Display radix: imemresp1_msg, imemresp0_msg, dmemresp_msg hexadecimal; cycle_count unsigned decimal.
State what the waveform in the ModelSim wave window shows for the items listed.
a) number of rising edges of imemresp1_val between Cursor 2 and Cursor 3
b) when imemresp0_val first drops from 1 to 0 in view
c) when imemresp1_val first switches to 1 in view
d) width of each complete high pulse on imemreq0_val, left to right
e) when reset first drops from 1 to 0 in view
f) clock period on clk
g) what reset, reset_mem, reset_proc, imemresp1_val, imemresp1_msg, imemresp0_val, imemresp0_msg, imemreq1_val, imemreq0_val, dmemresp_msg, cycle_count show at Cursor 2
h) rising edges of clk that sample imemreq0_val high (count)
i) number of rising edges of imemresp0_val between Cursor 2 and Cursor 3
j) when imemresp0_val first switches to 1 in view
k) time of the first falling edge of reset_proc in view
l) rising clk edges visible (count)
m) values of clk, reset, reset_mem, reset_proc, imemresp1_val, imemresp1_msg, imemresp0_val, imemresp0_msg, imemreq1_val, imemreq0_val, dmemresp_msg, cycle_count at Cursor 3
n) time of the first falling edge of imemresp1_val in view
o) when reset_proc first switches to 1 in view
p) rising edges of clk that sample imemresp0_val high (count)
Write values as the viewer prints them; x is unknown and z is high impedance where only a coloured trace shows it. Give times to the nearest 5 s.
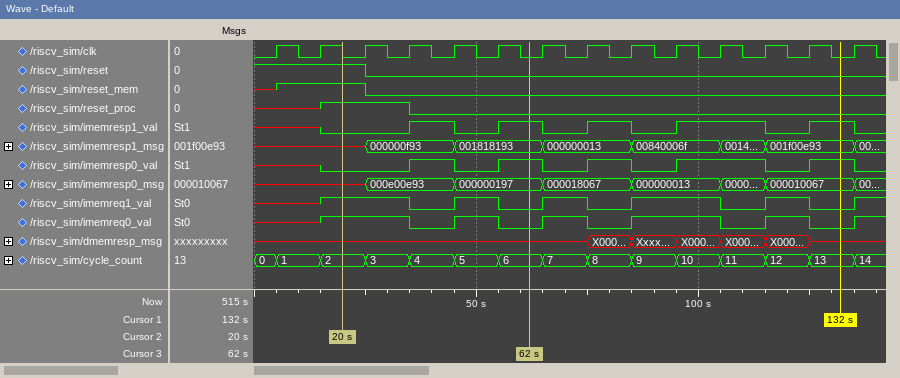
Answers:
2
45 s
35 s
10 s, 10 s, 20 s, 10 s
25 s
10 s
reset=1, reset_mem=1, reset_proc=1, imemresp1_val=0, imemresp1_msg=x, imemresp0_val=0, imemresp0_msg=x, imemreq1_val=1, imemreq0_val=1, dmemresp_msg=x, cycle_count=2
7
2
35 s
35 s
14
clk=0, reset=0, reset_mem=0, reset_proc=0, imemresp1_val=1, imemresp1_msg=001818193, imemresp0_val=1, imemresp0_msg=000000197, imemreq1_val=0, imemreq0_val=0, dmemresp_msg=x, cycle_count=6
45 s
15 s
6
